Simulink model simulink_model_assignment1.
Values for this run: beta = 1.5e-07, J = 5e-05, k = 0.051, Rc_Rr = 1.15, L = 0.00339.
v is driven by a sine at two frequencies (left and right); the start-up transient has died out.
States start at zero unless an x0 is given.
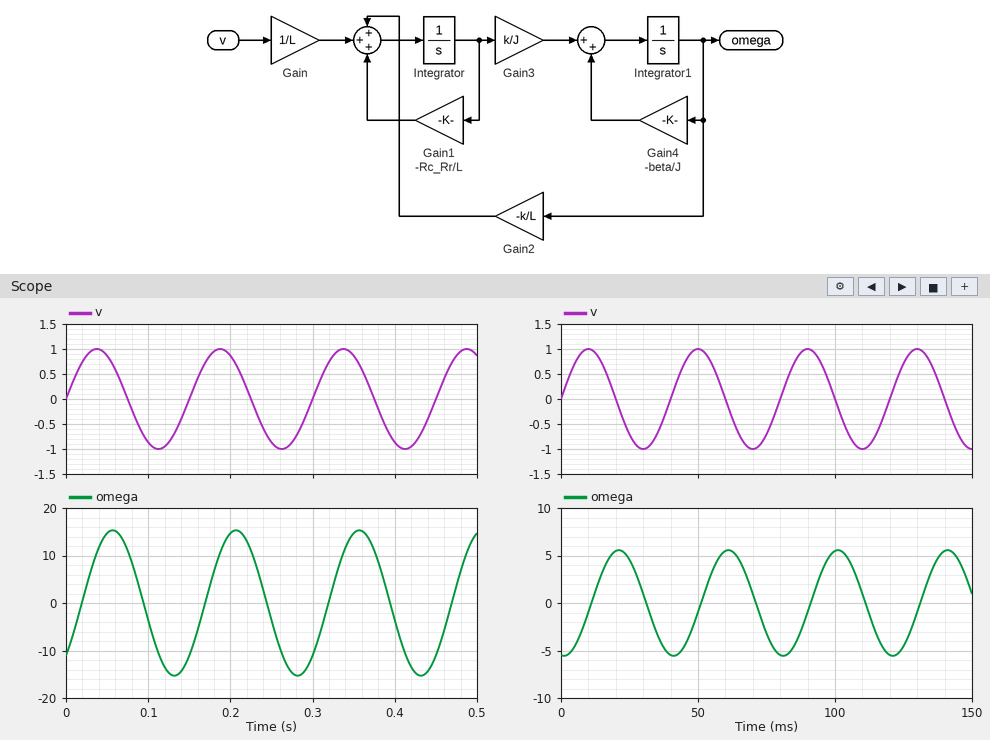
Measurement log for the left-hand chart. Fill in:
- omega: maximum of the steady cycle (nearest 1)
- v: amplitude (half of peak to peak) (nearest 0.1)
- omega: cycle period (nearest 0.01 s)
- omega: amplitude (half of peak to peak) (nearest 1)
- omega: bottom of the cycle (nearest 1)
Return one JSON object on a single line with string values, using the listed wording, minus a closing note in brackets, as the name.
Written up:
{"omega: maximum of the steady cycle": "15", "v: amplitude (half of peak to peak)": "1.0", "omega: cycle period": "0.15 s", "omega: amplitude (half of peak to peak)": "15", "omega: bottom of the cycle": "-15"}
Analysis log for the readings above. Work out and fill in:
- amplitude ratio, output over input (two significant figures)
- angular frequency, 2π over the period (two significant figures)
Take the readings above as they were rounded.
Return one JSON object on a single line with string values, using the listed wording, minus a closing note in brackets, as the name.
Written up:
{"amplitude ratio, output over input": "15", "angular frequency, 2π over the period": "42 rad/s"}
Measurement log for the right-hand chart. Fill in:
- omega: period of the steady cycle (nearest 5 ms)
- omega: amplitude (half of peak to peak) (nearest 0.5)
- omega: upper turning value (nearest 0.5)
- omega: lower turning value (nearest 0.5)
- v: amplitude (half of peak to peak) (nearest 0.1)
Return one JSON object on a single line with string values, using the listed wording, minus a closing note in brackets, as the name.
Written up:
{"omega: period of the steady cycle": "40 ms", "omega: amplitude (half of peak to peak)": "5.5", "omega: upper turning value": "5.5", "omega: lower turning value": "-5.5", "v: amplitude (half of peak to peak)": "1.0"}
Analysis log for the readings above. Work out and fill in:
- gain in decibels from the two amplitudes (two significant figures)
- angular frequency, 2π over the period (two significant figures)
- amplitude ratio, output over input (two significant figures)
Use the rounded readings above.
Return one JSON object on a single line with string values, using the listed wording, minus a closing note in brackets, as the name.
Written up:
{"gain in decibels from the two amplitudes": "15 dB", "angular frequency, 2π over the period": "0.16 rad/ms", "amplitude ratio, output over input": "5.5"}
